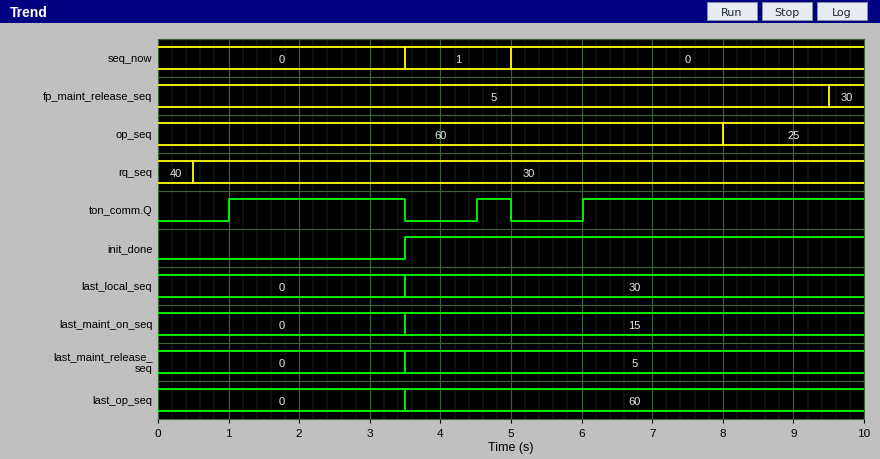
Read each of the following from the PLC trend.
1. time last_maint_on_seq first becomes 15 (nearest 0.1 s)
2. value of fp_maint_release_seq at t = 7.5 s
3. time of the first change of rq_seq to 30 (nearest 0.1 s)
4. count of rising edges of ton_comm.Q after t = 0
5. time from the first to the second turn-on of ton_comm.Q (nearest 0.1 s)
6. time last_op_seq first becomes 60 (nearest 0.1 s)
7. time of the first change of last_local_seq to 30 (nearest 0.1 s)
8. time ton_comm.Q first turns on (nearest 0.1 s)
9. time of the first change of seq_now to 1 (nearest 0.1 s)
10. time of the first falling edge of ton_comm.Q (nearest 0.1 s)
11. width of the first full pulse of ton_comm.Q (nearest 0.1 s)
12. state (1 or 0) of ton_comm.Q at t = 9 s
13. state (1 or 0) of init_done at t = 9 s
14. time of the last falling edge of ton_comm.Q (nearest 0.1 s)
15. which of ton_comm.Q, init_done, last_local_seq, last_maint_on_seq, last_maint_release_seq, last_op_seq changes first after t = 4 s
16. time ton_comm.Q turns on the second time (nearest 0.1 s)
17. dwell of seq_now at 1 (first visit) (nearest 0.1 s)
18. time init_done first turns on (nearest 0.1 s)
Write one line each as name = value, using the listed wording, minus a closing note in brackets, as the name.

time last_maint_on_seq first becomes 15 = 3.5 s
value of fp_maint_release_seq at t = 7.5 s = 5
time of the first change of rq_seq to 30 = 0.5 s
count of rising edges of ton_comm.Q after t = 0 = 3
time from the first to the second turn-on of ton_comm.Q = 3.5 s
time last_op_seq first becomes 60 = 3.5 s
time of the first change of last_local_seq to 30 = 3.5 s
time ton_comm.Q first turns on = 1.0 s
time of the first change of seq_now to 1 = 3.5 s
time of the first falling edge of ton_comm.Q = 3.5 s
width of the first full pulse of ton_comm.Q = 2.5 s
state (1 or 0) of ton_comm.Q at t = 9 s = 1
state (1 or 0) of init_done at t = 9 s = 1
time of the last falling edge of ton_comm.Q = 5.0 s
which of ton_comm.Q, init_done, last_local_seq, last_maint_on_seq, last_maint_release_seq, last_op_seq changes first after t = 4 s = ton_comm.Q
time ton_comm.Q turns on the second time = 4.5 s
dwell of seq_now at 1 (first visit) = 1.5 s
time init_done first turns on = 3.5 s
